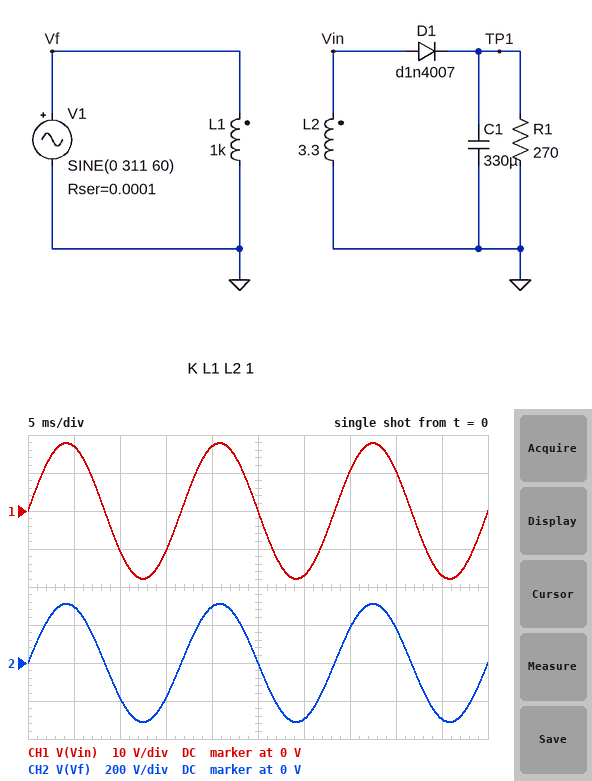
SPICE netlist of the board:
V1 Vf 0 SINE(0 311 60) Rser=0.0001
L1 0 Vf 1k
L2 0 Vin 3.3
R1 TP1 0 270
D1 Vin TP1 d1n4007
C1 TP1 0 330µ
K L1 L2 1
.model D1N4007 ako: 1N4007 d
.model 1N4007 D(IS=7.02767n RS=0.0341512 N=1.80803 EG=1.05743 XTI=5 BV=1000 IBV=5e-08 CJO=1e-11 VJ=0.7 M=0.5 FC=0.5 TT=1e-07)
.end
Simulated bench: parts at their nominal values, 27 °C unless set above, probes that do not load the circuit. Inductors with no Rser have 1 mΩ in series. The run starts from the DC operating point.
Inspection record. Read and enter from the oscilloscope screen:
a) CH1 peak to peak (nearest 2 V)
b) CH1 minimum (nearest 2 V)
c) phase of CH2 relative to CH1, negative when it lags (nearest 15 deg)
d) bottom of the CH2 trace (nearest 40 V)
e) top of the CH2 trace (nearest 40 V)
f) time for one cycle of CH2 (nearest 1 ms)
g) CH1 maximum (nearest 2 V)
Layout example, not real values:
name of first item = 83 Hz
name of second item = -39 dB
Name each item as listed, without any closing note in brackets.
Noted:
CH1 peak to peak = 36 V
CH1 minimum = -18 V
phase of CH2 relative to CH1, negative when it lags = 0 deg
bottom of the CH2 trace = -320 V
top of the CH2 trace = 320 V
time for one cycle of CH2 = 17 ms
CH1 maximum = 18 V
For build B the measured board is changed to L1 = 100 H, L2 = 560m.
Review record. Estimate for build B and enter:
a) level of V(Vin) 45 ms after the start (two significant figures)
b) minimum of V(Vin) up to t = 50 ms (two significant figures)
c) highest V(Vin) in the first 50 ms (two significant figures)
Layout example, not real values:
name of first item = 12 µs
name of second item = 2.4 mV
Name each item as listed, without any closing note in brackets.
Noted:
level of V(Vin) 45 ms after the start = -22 V
minimum of V(Vin) up to t = 50 ms = -23 V
highest V(Vin) in the first 50 ms = 23 V
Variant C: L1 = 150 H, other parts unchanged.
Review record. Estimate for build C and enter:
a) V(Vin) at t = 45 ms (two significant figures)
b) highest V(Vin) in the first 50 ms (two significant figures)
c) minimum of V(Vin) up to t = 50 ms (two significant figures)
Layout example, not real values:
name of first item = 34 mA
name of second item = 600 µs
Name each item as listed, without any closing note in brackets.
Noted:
V(Vin) at t = 45 ms = -44 V
highest V(Vin) in the first 50 ms = 46 V
minimum of V(Vin) up to t = 50 ms = -46 V
